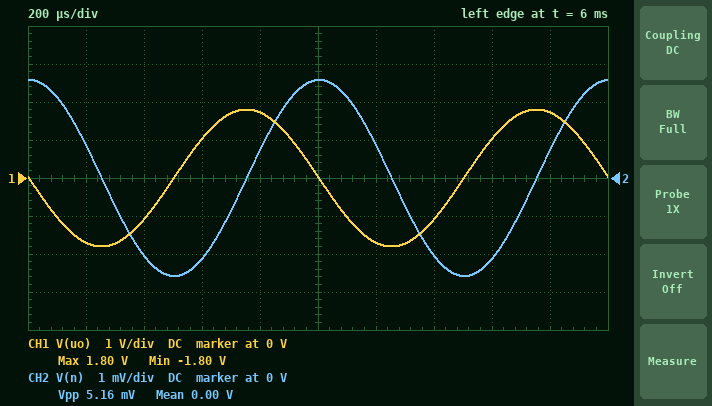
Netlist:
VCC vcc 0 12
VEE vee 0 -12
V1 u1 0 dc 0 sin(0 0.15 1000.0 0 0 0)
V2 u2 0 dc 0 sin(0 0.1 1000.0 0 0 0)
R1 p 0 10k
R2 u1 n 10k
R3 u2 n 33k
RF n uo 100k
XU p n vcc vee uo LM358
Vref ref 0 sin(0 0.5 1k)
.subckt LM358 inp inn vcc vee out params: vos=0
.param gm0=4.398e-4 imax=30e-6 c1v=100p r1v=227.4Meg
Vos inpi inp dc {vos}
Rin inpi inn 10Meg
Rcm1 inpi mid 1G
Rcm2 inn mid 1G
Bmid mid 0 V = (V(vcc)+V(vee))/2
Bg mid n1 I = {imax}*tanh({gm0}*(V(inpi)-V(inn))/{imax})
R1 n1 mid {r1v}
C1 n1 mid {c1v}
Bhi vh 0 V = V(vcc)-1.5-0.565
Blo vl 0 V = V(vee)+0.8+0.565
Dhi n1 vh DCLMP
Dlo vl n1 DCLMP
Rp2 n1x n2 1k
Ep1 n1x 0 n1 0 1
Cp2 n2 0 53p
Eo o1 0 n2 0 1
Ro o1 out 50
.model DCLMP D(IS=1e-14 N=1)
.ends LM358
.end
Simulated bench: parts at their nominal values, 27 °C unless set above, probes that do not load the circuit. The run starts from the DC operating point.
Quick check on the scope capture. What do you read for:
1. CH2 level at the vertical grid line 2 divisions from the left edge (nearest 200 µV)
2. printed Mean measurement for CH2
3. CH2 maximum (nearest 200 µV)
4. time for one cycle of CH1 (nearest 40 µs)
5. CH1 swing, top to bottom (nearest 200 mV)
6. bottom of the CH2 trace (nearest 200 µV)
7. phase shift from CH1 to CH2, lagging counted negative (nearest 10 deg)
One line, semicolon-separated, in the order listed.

-2.0 mV; 0.00 V; 2.6 mV; 1.00 ms; 3.6 V; -2.6 mV; -90 deg
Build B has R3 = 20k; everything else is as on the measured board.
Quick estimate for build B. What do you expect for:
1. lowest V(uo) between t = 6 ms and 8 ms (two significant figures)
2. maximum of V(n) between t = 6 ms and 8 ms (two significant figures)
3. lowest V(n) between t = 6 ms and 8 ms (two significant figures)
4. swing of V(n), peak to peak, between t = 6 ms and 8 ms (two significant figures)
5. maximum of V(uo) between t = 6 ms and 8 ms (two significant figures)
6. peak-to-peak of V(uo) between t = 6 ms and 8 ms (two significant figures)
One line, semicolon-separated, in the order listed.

-2.0 V; 2.9 mV; -2.9 mV; 5.7 mV; 2.0 V; 4.0 V
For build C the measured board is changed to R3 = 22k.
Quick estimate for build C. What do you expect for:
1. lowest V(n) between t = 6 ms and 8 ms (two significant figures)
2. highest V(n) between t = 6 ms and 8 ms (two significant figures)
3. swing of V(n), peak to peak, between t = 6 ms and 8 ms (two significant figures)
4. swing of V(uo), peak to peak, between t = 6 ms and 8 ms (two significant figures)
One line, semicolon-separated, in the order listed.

-2.8 mV; 2.8 mV; 5.6 mV; 3.9 V
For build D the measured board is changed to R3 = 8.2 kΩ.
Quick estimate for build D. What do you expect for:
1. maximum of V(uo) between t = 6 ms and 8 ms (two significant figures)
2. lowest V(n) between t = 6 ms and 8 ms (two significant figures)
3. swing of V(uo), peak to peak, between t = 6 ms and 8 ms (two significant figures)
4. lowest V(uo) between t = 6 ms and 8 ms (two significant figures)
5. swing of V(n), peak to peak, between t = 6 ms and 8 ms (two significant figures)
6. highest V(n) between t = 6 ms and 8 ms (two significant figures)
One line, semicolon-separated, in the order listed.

2.7 V; -3.9 mV; 5.4 V; -2.7 V; 7.8 mV; 3.9 mV
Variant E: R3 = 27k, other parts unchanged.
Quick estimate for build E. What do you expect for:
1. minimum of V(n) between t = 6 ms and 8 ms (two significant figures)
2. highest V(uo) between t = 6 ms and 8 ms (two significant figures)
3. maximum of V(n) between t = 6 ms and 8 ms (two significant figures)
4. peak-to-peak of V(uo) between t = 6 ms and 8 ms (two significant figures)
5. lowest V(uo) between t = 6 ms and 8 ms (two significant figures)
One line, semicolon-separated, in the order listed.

-2.7 mV; 1.9 V; 2.7 mV; 3.7 V; -1.9 V
